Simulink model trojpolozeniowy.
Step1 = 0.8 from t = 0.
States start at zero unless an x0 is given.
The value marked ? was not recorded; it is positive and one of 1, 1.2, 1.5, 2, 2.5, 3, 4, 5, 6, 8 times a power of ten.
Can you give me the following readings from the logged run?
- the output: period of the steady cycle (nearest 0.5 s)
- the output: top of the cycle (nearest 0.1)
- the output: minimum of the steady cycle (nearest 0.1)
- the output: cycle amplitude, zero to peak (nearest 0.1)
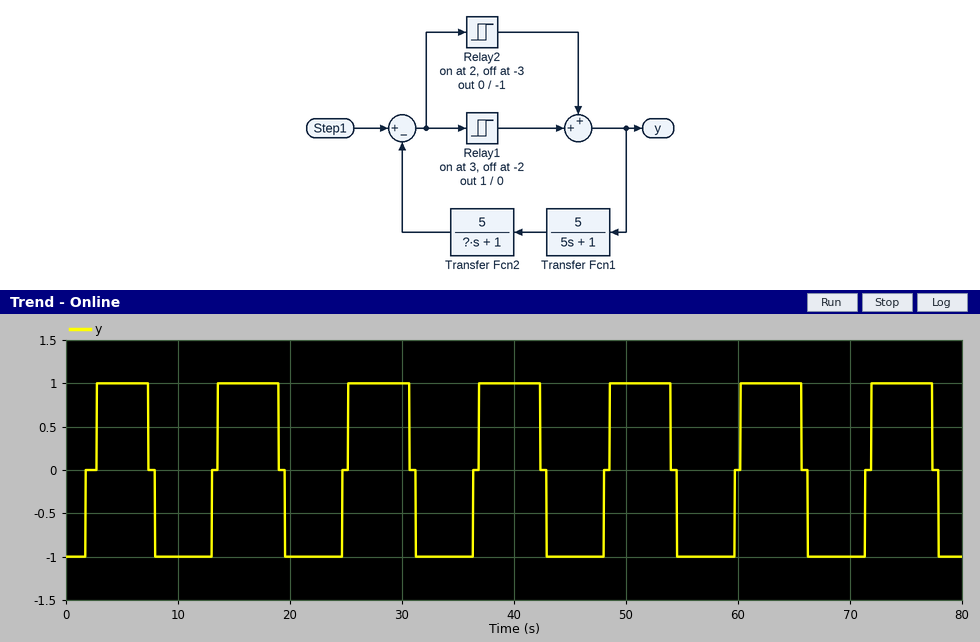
11.5 s
1.0
-1.0
1.0
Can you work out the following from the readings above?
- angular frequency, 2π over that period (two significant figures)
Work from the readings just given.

0.55 rad/s
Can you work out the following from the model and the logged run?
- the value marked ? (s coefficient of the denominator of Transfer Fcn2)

5
